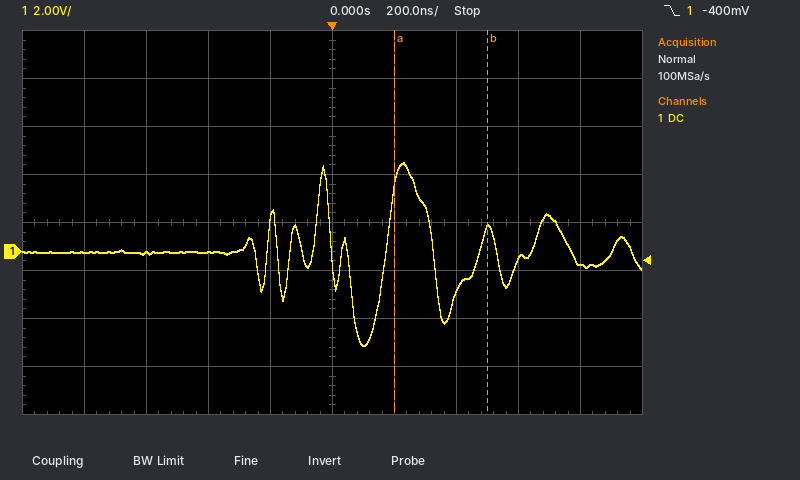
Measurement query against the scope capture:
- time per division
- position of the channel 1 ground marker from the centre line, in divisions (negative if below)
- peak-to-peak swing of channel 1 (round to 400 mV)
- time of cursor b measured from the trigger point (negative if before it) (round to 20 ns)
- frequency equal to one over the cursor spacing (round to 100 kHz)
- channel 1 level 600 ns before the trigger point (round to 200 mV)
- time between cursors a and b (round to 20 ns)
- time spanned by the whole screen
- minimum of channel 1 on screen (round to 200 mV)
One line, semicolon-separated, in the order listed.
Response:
200 ns; -0.6 div; 7.6 V; +500 ns; 3.3 MHz; 0.0 V; 300 ns; 2 µs; -4.0 V
